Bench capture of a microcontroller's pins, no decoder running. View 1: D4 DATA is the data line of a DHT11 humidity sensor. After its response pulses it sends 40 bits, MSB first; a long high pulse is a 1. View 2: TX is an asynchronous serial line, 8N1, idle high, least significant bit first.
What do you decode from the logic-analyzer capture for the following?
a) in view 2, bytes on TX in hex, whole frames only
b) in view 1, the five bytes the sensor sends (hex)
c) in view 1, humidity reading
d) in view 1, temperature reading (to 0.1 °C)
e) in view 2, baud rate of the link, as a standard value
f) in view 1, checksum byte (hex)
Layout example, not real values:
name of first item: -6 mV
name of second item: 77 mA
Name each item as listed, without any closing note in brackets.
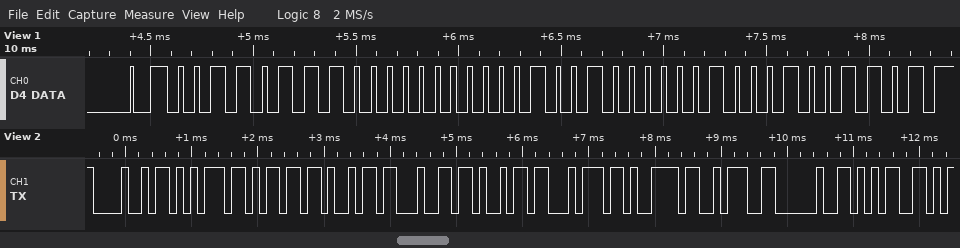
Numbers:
in view 2, bytes on TX in hex, whole frames only: 0x48 0x75 0x6D 0x69 0x64 0x69 0x74 0x79 0x3A 0x20 0x35
in view 1, the five bytes the sensor sends: 37 00 12 04 4D
in view 1, humidity reading: 55 %
in view 1, temperature reading: 18.4 °C
in view 2, baud rate of the link, as a standard value: 9600 baud
in view 1, checksum byte: 0x4D
